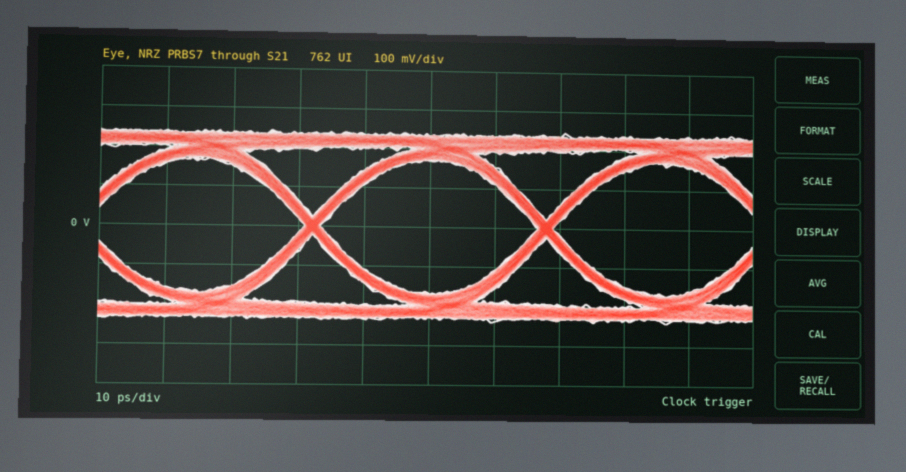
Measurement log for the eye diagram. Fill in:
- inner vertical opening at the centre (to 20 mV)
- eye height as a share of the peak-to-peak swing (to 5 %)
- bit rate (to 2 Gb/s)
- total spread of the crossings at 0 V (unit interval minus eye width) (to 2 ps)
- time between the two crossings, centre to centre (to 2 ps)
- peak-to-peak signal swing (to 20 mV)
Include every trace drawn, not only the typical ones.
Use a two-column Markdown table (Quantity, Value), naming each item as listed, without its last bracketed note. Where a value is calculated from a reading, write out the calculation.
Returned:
| Quantity | Value |
|---|---|
| inner vertical opening at the centre | 340 mV |
| eye height as a share of the peak-to-peak swing | 340 mV / 480 mV ≈ 70.8 %, so 70 % to the nearest 5 % |
| bit rate | 28 Gb/s |
| total spread of the crossings at 0 V (unit interval minus eye width) | 2 ps |
| time between the two crossings, centre to centre | 36 ps |
| peak-to-peak signal swing | 480 mV |
